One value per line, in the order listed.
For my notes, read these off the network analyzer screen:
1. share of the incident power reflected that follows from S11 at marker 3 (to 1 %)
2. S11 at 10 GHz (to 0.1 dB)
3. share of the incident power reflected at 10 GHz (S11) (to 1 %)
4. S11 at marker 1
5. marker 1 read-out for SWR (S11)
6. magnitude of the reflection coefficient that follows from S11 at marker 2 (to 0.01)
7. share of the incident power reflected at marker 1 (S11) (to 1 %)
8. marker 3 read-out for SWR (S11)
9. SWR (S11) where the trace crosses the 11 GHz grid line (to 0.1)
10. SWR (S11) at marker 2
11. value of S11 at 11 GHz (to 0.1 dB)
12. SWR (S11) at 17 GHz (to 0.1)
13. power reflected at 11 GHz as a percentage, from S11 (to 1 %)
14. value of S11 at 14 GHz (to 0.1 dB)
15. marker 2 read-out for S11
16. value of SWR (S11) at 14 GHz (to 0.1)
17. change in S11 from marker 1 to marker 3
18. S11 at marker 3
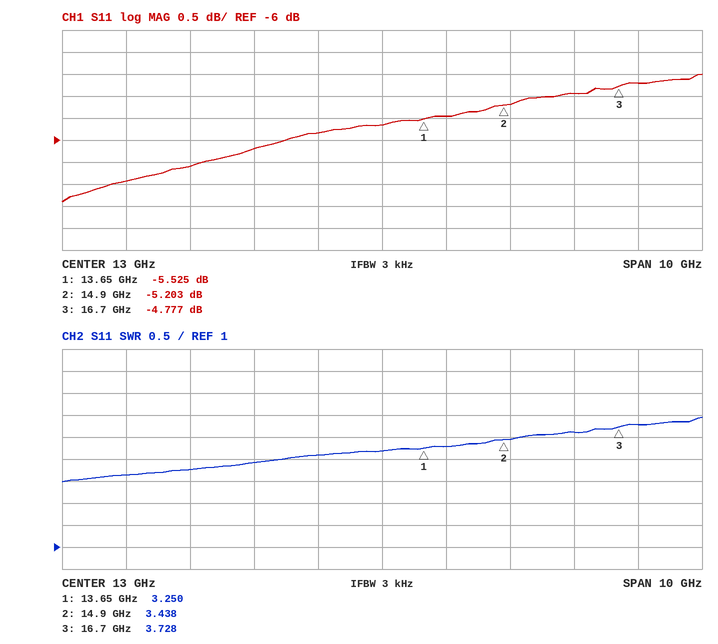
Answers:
33 %
-6.6 dB
22 %
-5.525 dB
3.250
0.55
28 %
3.728
2.9
3.438
-6.2 dB
3.8
24 %
-5.5 dB
-5.203 dB
3.3
0.748 dB
-4.777 dB
